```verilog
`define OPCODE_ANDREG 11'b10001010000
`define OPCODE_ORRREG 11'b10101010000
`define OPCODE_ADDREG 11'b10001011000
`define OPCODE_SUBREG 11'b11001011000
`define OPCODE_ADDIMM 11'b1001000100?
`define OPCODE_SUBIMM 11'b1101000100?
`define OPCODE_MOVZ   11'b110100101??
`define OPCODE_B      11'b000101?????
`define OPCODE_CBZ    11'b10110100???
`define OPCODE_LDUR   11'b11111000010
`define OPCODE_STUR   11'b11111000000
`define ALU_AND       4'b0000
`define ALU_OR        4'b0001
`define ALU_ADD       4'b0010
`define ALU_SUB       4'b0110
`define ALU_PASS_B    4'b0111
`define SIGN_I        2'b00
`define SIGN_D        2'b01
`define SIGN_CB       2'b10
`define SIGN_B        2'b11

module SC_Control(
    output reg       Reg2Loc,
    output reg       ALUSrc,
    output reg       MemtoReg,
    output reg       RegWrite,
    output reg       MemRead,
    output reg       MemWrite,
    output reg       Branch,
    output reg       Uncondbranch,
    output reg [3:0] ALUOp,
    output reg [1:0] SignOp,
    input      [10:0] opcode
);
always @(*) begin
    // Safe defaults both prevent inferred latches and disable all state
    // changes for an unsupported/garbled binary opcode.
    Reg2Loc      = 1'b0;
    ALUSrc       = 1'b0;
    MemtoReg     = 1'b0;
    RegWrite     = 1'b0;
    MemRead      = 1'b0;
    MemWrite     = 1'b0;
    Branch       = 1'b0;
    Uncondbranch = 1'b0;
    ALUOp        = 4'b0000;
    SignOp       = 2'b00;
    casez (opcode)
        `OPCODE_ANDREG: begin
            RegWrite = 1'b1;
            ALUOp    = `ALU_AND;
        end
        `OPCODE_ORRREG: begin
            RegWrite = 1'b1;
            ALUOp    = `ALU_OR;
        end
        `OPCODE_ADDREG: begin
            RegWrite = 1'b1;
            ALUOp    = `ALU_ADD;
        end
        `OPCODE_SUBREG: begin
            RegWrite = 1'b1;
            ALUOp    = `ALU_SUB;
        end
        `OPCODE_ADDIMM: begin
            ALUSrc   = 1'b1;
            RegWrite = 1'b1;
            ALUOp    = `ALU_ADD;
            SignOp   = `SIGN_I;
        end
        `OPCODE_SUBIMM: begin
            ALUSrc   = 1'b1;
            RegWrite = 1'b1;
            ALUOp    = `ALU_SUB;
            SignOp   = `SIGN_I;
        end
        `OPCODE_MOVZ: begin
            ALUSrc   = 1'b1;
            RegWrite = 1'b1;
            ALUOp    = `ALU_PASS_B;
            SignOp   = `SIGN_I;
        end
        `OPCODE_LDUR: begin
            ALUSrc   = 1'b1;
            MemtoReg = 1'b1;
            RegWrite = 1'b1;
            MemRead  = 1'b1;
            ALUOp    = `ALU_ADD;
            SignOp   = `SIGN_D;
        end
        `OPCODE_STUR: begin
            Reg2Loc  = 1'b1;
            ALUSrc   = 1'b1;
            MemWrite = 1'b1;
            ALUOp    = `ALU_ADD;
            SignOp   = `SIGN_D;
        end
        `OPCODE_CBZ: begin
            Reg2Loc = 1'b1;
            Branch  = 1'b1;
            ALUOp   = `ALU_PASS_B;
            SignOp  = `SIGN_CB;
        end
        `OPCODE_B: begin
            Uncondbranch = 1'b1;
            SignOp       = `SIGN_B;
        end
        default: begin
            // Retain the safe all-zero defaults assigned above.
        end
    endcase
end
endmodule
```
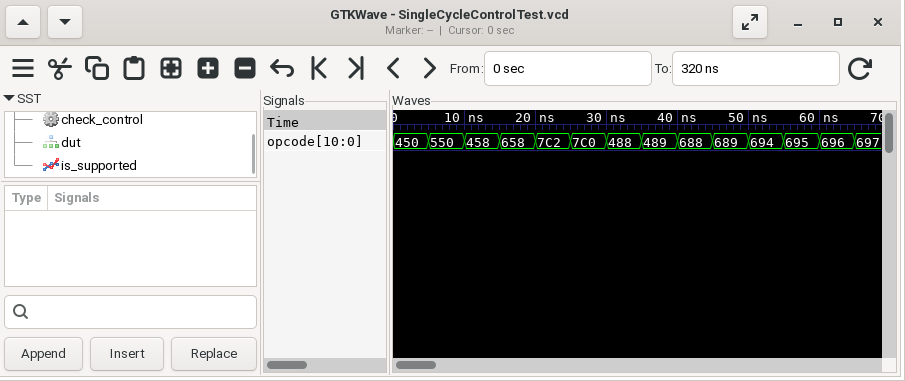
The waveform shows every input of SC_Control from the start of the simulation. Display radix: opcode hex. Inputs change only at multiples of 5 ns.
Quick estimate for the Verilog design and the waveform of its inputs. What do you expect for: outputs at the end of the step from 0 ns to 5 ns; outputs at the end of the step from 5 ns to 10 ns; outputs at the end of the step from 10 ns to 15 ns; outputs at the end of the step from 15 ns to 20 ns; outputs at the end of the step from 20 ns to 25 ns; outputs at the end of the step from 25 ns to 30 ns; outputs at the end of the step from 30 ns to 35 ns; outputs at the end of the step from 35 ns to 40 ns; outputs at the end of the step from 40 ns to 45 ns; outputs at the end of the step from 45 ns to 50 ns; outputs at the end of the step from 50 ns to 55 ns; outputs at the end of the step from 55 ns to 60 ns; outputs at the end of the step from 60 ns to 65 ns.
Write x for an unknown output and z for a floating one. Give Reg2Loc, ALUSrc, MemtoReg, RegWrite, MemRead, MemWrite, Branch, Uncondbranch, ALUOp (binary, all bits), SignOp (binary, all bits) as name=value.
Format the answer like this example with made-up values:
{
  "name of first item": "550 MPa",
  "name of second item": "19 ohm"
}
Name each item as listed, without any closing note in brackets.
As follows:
{
  "outputs at the end of the step from 0 ns to 5 ns": "Reg2Loc=0, ALUSrc=0, MemtoReg=0, RegWrite=1, MemRead=0, MemWrite=0, Branch=0, Uncondbranch=0, ALUOp=0000, SignOp=00",
  "outputs at the end of the step from 5 ns to 10 ns": "Reg2Loc=0, ALUSrc=0, MemtoReg=0, RegWrite=1, MemRead=0, MemWrite=0, Branch=0, Uncondbranch=0, ALUOp=0001, SignOp=00",
  "outputs at the end of the step from 10 ns to 15 ns": "Reg2Loc=0, ALUSrc=0, MemtoReg=0, RegWrite=1, MemRead=0, MemWrite=0, Branch=0, Uncondbranch=0, ALUOp=0010, SignOp=00",
  "outputs at the end of the step from 15 ns to 20 ns": "Reg2Loc=0, ALUSrc=0, MemtoReg=0, RegWrite=1, MemRead=0, MemWrite=0, Branch=0, Uncondbranch=0, ALUOp=0110, SignOp=00",
  "outputs at the end of the step from 20 ns to 25 ns": "Reg2Loc=0, ALUSrc=1, MemtoReg=1, RegWrite=1, MemRead=1, MemWrite=0, Branch=0, Uncondbranch=0, ALUOp=0010, SignOp=01",
  "outputs at the end of the step from 25 ns to 30 ns": "Reg2Loc=1, ALUSrc=1, MemtoReg=0, RegWrite=0, MemRead=0, MemWrite=1, Branch=0, Uncondbranch=0, ALUOp=0010, SignOp=01",
  "outputs at the end of the step from 30 ns to 35 ns": "Reg2Loc=0, ALUSrc=1, MemtoReg=0, RegWrite=1, MemRead=0, MemWrite=0, Branch=0, Uncondbranch=0, ALUOp=0010, SignOp=00",
  "outputs at the end of the step from 35 ns to 40 ns": "Reg2Loc=0, ALUSrc=1, MemtoReg=0, RegWrite=1, MemRead=0, MemWrite=0, Branch=0, Uncondbranch=0, ALUOp=0010, SignOp=00",
  "outputs at the end of the step from 40 ns to 45 ns": "Reg2Loc=0, ALUSrc=1, MemtoReg=0, RegWrite=1, MemRead=0, MemWrite=0, Branch=0, Uncondbranch=0, ALUOp=0110, SignOp=00",
  "outputs at the end of the step from 45 ns to 50 ns": "Reg2Loc=0, ALUSrc=1, MemtoReg=0, RegWrite=1, MemRead=0, MemWrite=0, Branch=0, Uncondbranch=0, ALUOp=0110, SignOp=00",
  "outputs at the end of the step from 50 ns to 55 ns": "Reg2Loc=0, ALUSrc=1, MemtoReg=0, RegWrite=1, MemRead=0, MemWrite=0, Branch=0, Uncondbranch=0, ALUOp=0111, SignOp=00",
  "outputs at the end of the step from 55 ns to 60 ns": "Reg2Loc=0, ALUSrc=1, MemtoReg=0, RegWrite=1, MemRead=0, MemWrite=0, Branch=0, Uncondbranch=0, ALUOp=0111, SignOp=00",
  "outputs at the end of the step from 60 ns to 65 ns": "Reg2Loc=0, ALUSrc=1, MemtoReg=0, RegWrite=1, MemRead=0, MemWrite=0, Branch=0, Uncondbranch=0, ALUOp=0111, SignOp=00"
}
